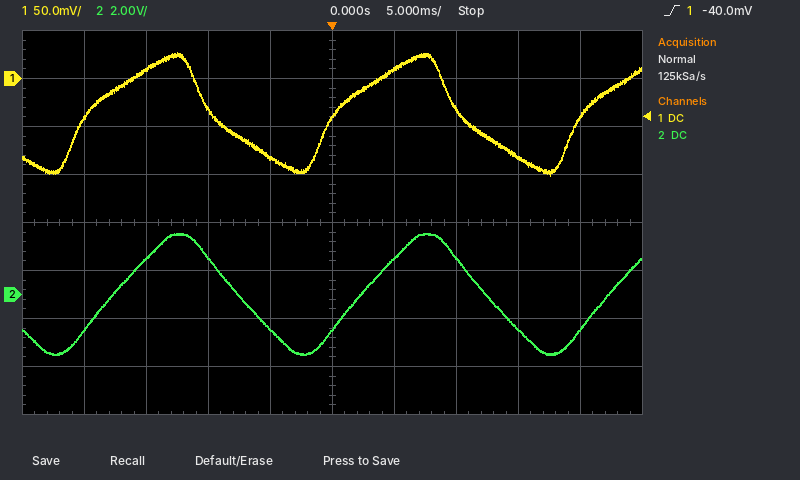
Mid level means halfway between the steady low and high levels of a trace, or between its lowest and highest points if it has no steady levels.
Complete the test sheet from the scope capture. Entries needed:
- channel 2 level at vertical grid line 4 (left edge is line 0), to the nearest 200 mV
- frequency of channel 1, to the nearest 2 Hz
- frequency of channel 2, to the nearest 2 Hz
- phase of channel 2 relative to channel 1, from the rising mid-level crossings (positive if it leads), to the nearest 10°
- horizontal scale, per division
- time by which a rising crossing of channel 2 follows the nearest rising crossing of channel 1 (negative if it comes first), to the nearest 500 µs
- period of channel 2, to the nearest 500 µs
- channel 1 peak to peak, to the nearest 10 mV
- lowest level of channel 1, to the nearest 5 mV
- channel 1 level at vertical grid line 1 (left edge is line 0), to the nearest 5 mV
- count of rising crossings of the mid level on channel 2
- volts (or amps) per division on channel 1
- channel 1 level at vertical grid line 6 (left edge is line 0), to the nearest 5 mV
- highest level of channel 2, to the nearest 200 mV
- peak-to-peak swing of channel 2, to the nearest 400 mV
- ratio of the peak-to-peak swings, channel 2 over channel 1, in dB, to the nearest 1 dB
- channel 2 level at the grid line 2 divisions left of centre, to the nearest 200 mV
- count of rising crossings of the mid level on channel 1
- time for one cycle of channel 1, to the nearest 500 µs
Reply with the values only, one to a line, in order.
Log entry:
-1.4 V
50 Hz
50 Hz
-40°
5 ms
+2.0 ms
20.0 ms
130 mV
-100 mV
-40 mV
3
50 mV
10 mV
2.6 V
5.2 V
32 dB
1.6 V
3
20.0 ms
